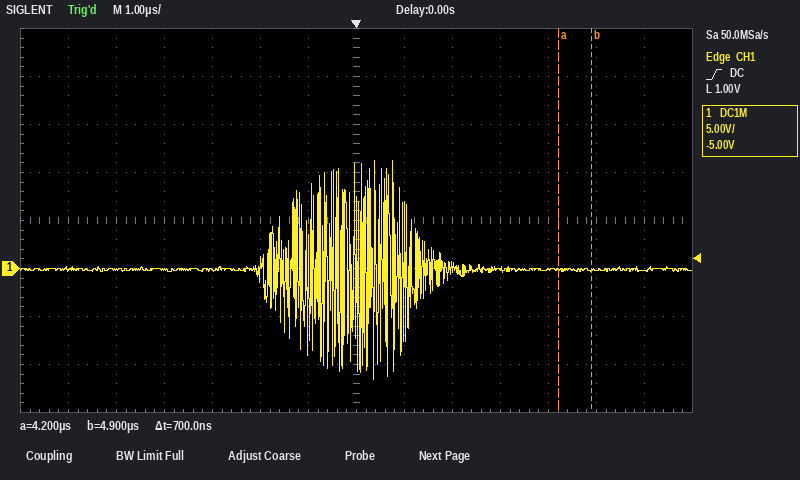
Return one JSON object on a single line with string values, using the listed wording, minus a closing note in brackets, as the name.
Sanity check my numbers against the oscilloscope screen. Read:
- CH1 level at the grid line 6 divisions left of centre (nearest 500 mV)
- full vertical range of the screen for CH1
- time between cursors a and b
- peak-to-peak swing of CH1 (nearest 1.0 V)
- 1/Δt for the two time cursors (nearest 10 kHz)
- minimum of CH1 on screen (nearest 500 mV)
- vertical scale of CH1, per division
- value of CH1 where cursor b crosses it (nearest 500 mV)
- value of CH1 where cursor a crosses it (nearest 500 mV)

{"CH1 level at the grid line 6 divisions left of centre": "0.0 V", "full vertical range of the screen for CH1": "40 V", "time between cursors a and b": "700 ns", "peak-to-peak swing of CH1": "23.0 V", "1/Δt for the two time cursors": "1.43 MHz", "minimum of CH1 on screen": "-11.5 V", "vertical scale of CH1, per division": "5 V", "value of CH1 where cursor b crosses it": "0.0 V", "value of CH1 where cursor a crosses it": "0.0 V"}
